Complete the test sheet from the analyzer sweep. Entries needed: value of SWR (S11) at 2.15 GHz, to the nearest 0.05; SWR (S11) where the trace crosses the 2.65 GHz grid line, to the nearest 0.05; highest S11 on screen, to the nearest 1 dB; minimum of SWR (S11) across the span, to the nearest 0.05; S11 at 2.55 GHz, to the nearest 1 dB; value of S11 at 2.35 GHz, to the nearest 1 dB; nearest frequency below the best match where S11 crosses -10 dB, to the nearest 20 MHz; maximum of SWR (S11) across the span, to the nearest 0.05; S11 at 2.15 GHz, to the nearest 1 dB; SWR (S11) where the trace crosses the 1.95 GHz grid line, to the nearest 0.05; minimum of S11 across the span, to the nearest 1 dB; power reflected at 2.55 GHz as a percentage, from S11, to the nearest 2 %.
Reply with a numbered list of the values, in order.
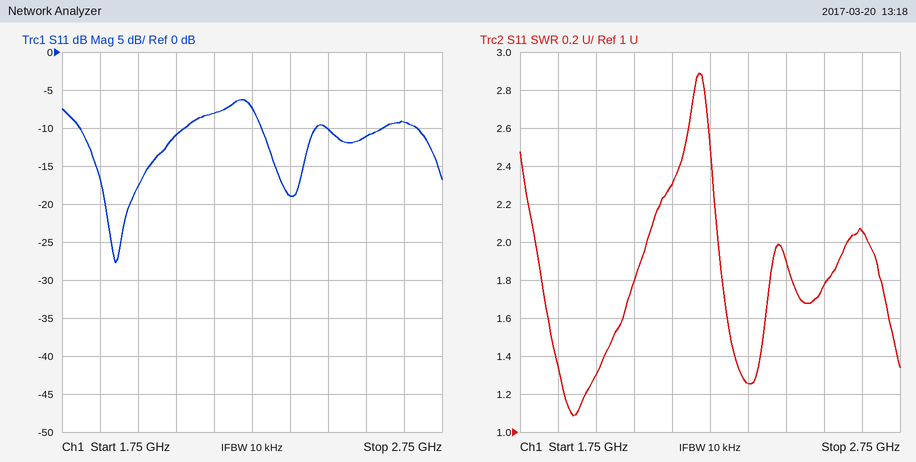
1. 2.30
2. 2.05
3. -6 dB
4. 1.10
5. -11 dB
6. -19 dB
7. 1.80 GHz
8. 2.90
9. -8 dB
10. 1.30
11. -28 dB
12. 8 %
